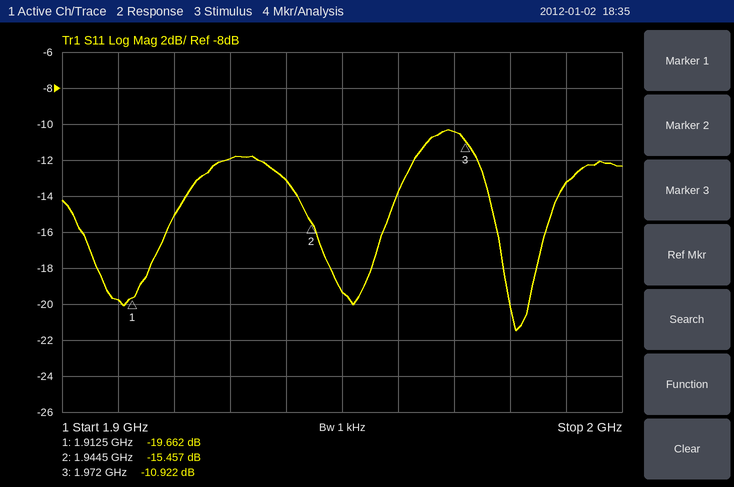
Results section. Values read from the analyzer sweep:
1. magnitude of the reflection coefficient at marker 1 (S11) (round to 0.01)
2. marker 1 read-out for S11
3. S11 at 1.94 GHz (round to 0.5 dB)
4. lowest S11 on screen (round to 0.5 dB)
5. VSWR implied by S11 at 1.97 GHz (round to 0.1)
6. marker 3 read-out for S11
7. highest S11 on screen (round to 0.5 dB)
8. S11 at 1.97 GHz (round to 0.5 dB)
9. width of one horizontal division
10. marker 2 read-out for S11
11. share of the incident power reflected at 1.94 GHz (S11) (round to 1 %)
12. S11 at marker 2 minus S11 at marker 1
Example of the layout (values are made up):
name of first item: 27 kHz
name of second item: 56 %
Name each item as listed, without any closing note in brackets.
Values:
magnitude of the reflection coefficient at marker 1 (S11): 0.10
marker 1 read-out for S11: -19.662 dB
S11 at 1.94 GHz: -13.0 dB
lowest S11 on screen: -21.5 dB
VSWR implied by S11 at 1.97 GHz: 1.9
marker 3 read-out for S11: -10.922 dB
highest S11 on screen: -10.5 dB
S11 at 1.97 GHz: -10.5 dB
width of one horizontal division: 10 MHz
marker 2 read-out for S11: -15.457 dB
share of the incident power reflected at 1.94 GHz (S11): 5 %
S11 at marker 2 minus S11 at marker 1: 4.205 dB
